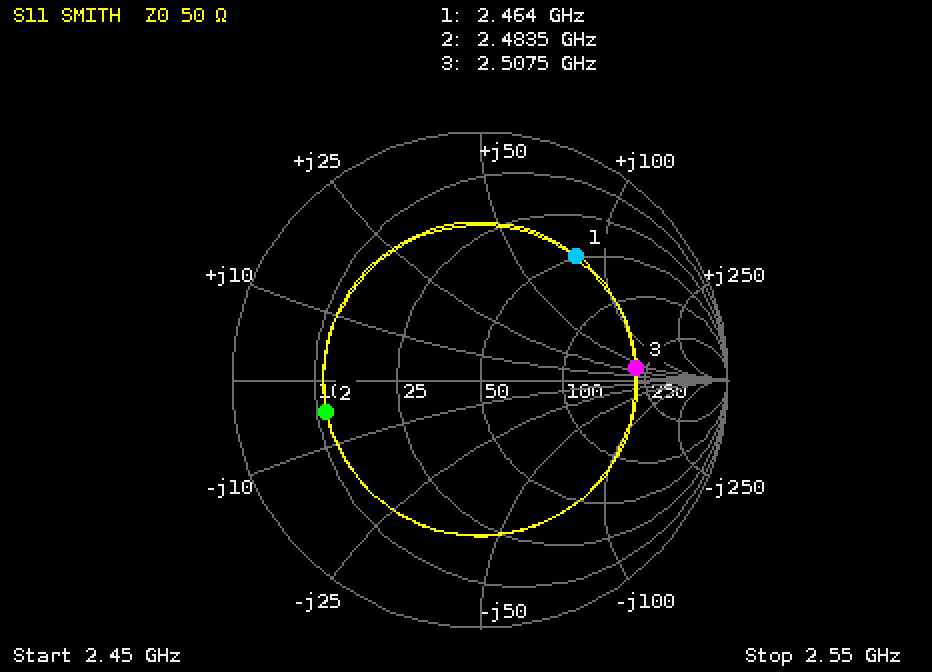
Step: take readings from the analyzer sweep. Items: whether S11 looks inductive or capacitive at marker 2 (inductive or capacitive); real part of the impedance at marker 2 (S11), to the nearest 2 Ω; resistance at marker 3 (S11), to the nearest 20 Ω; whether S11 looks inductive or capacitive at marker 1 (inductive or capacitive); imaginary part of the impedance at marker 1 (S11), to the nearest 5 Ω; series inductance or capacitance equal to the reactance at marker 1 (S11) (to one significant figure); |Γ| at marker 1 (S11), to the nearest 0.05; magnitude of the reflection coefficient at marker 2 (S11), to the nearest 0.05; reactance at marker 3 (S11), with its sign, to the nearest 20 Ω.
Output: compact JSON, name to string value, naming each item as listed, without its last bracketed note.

{"whether S11 looks inductive or capacitive at marker 2": "capacitive", "real part of the impedance at marker 2 (S11), to the nearest 2 Ω": "12 Ω", "resistance at marker 3 (S11), to the nearest 20 Ω": "220 Ω", "whether S11 looks inductive or capacitive at marker 1": "inductive", "imaginary part of the impedance at marker 1 (S11), to the nearest 5 Ω": "+80 Ω", "series inductance or capacitance equal to the reactance at marker 1 (S11)": "5 nH", "|Γ| at marker 1 (S11), to the nearest 0.05": "0.65", "magnitude of the reflection coefficient at marker 2 (S11), to the nearest 0.05": "0.65", "reactance at marker 3 (S11), with its sign, to the nearest 20 Ω": "+40 Ω"}
